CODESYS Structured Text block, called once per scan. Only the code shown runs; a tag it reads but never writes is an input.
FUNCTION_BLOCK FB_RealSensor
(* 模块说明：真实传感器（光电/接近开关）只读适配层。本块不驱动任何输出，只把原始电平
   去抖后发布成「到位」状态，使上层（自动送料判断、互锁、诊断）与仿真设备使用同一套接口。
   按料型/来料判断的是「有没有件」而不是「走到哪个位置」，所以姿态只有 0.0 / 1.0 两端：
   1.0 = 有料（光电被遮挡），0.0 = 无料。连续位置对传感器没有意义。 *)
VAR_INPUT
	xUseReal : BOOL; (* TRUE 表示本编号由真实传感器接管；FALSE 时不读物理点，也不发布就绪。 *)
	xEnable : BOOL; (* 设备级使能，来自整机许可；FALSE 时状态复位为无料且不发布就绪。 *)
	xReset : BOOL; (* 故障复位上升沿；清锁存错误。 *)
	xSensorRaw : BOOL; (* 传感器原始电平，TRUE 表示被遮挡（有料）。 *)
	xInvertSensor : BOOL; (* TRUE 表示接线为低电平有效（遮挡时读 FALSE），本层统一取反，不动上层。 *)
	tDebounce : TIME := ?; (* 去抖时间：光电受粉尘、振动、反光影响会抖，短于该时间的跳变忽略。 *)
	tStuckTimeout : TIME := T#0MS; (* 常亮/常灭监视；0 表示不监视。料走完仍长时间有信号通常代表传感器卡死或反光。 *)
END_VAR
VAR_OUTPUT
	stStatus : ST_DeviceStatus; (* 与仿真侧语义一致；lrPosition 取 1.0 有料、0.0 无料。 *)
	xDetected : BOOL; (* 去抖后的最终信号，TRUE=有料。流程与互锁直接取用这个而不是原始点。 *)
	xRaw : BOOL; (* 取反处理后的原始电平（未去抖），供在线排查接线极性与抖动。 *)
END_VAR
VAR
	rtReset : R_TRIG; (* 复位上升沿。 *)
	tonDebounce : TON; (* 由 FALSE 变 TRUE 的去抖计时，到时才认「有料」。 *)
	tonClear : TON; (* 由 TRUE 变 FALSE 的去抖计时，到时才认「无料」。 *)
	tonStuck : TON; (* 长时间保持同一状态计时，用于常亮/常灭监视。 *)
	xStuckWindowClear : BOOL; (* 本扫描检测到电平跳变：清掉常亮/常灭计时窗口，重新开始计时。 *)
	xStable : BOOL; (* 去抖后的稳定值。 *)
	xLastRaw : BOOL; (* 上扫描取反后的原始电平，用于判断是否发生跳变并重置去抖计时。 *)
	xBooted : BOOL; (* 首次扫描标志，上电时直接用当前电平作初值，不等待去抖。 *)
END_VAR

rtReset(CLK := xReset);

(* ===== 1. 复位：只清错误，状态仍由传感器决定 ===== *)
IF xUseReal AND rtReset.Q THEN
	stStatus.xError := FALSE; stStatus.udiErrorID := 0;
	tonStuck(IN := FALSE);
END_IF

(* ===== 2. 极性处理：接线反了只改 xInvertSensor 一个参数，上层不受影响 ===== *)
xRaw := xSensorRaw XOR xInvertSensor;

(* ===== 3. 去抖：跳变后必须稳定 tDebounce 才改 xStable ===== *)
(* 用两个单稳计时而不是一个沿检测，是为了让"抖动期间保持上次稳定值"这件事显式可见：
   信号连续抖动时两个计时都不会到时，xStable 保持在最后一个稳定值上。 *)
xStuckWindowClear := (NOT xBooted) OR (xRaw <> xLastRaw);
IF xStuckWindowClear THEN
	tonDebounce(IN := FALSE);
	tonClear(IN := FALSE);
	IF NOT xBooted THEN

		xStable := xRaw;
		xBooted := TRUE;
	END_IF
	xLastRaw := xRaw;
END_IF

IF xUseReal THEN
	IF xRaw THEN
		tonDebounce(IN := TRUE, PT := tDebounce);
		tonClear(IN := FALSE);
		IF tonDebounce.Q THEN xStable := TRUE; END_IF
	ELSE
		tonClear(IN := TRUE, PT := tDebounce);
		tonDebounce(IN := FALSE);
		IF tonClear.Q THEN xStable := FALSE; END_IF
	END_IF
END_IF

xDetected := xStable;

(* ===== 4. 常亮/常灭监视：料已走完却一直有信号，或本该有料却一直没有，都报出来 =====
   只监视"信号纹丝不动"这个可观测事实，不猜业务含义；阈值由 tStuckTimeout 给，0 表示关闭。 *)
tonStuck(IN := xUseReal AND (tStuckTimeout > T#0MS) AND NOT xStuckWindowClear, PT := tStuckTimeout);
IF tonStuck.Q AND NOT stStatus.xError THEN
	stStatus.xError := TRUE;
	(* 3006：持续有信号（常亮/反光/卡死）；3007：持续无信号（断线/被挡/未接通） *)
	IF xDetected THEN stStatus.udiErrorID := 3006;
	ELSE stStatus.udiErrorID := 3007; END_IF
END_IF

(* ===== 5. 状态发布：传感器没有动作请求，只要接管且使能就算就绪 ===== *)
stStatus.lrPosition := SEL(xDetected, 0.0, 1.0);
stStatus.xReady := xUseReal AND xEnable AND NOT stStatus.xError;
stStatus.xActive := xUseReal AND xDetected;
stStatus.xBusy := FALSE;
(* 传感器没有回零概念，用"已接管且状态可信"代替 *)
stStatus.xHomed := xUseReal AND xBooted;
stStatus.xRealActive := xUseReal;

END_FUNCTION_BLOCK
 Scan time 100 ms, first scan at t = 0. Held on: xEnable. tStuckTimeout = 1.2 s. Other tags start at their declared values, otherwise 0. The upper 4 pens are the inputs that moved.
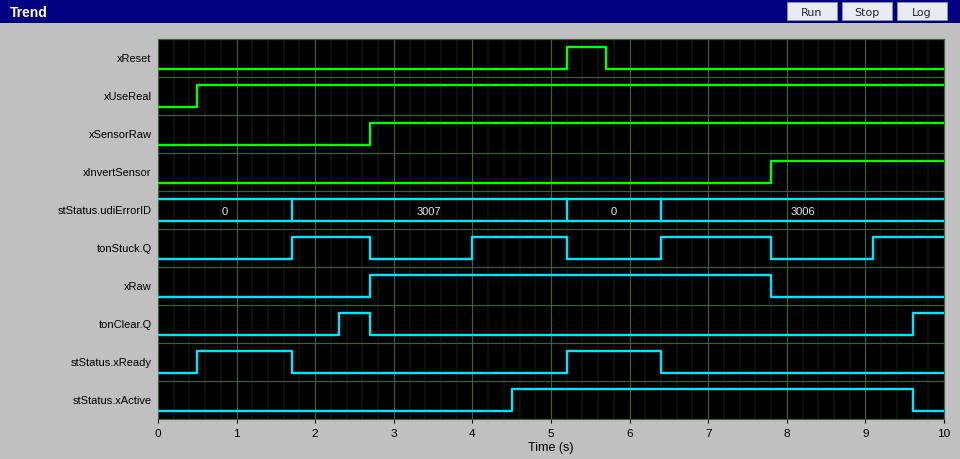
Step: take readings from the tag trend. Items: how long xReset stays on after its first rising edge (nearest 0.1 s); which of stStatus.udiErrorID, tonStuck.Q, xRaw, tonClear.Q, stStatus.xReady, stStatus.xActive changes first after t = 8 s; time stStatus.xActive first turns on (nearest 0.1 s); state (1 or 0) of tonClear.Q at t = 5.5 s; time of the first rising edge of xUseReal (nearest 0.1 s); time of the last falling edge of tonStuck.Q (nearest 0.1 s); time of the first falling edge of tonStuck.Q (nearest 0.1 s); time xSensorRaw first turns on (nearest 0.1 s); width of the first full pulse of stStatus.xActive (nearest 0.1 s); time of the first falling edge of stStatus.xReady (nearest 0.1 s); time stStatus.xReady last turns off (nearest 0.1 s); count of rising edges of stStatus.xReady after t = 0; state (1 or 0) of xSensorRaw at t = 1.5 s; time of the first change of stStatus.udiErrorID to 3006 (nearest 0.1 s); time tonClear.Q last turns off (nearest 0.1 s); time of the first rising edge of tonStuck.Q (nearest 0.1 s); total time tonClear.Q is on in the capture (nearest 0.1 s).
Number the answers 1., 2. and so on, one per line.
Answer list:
1. 0.5 s
2. tonStuck.Q
3. 4.5 s
4. 0
5. 0.5 s
6. 7.8 s
7. 2.7 s
8. 2.7 s
9. 5.1 s
10. 1.7 s
11. 6.4 s
12. 2
13. 0
14. 6.4 s
15. 2.7 s
16. 1.7 s
17. 0.8 s
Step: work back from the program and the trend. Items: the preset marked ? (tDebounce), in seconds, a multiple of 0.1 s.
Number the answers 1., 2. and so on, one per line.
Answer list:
1. 1.8 s
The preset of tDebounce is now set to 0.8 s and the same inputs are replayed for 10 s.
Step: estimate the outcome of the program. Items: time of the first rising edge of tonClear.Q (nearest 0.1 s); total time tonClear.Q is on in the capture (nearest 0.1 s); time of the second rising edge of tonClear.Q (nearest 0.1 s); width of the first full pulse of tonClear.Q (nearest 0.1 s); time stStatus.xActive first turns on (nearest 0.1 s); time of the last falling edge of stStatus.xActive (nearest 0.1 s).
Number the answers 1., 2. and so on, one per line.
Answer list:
1. 1.3 s
2. 2.8 s
3. 8.6 s
4. 1.4 s
5. 3.5 s
6. 8.6 s
